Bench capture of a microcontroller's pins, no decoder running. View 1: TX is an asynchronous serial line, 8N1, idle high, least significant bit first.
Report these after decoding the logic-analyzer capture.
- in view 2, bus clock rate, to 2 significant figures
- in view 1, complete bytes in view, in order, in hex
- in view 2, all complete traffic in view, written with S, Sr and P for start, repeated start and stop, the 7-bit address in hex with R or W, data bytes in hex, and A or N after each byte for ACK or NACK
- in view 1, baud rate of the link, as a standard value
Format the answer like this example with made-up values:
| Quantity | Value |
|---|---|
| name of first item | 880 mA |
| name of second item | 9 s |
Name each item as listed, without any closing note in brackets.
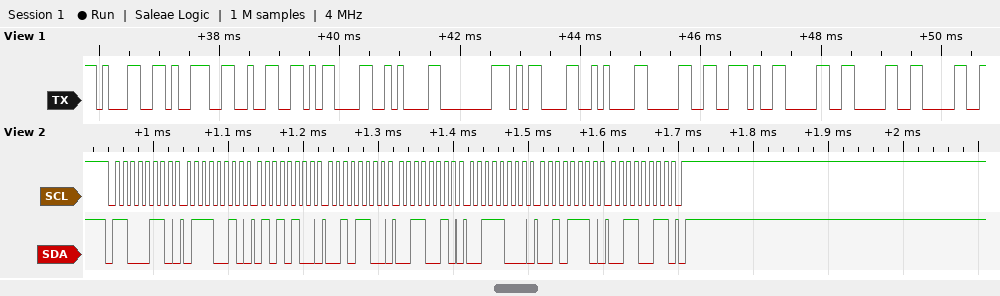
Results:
| Quantity | Value |
|---|---|
| in view 2, bus clock rate, to 2 significant figures | 100 kHz |
| in view 1, complete bytes in view, in order, in hex | 31 39 32 0D 0A 80 0D 0A 30 2E 30 30 30 |
| in view 2, all complete traffic in view, written with S, Sr and P for start, repeated start and stop, the 7-bit address in hex with R or W, data bytes in hex, and A or N after each byte for ACK or NACK | S 63W A 72 A 54 A 2C A 32 A 38 A 2E A 33 A P |
| in view 1, baud rate of the link, as a standard value | 9600 baud |
